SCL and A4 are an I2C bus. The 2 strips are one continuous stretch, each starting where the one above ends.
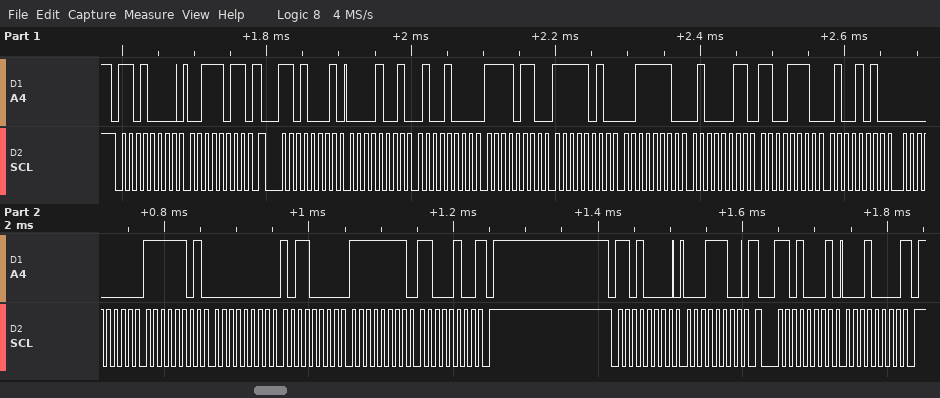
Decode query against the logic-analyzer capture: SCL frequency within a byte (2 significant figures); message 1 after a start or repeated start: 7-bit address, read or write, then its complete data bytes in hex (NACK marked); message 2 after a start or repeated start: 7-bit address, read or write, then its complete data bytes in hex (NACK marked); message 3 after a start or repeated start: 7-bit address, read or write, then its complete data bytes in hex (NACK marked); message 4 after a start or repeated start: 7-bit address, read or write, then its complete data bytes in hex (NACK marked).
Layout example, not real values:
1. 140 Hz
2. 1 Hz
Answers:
1. 100 kHz
2. 0x68 write: 3B
3. 0x68 read: 09 48 F6 FA 3E 43 CE 4A 00 FD 00 B0 FF C4 NACK
4. 0x68 write: 1C
5. 0x68 read: 10 NACK
